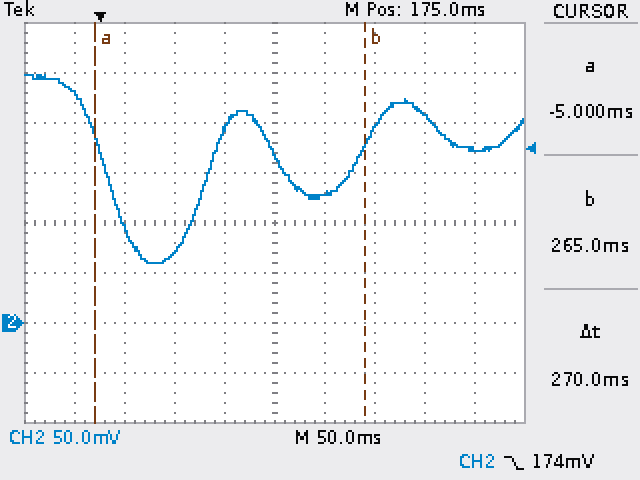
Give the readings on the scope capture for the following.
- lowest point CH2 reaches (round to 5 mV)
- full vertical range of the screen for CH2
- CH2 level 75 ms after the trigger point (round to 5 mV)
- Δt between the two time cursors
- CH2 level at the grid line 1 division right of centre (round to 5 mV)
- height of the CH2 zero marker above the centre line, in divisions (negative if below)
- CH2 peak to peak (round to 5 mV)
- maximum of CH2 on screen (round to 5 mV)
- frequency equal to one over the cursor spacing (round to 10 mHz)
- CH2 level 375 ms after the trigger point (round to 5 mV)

60 mV
400 mV
70 mV
270 ms
130 mV
-2.0 div
190 mV
250 mV
3.70 Hz
175 mV
